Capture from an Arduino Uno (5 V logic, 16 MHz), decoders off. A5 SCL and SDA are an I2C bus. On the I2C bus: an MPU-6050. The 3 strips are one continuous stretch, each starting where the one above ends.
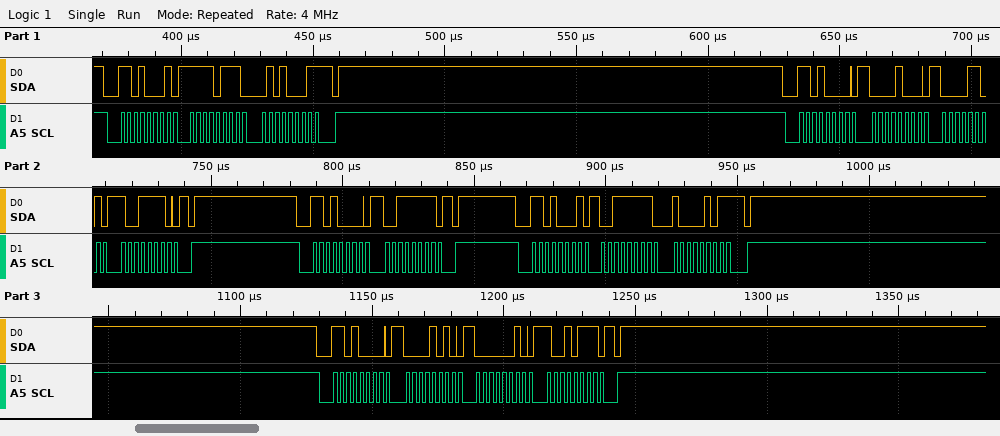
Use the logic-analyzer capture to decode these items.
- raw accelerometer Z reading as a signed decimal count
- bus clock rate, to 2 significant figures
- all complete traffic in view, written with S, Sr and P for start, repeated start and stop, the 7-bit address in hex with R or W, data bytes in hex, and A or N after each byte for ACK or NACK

16261
400 kHz
S 68R A F7 A 51 N P S 68W A 08 A 0D A 9E A P S 68W A 3F A P S 68R A 3F A 85 N P S 68W A 0A A 02 A 97 A P
